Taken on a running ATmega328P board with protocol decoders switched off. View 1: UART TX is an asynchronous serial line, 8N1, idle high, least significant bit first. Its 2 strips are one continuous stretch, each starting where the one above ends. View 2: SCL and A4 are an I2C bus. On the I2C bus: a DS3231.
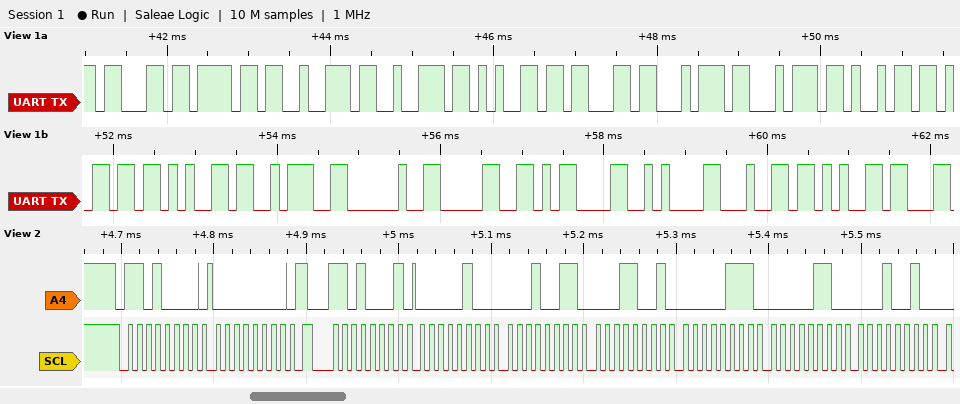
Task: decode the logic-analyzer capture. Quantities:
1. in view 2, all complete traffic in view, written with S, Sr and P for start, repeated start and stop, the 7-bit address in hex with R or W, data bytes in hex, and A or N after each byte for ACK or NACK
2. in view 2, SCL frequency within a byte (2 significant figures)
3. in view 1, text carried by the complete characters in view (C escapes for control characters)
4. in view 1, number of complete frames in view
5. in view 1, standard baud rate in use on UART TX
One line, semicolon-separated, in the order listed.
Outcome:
S 68W A 00 A Sr 68R A 04 A 13 A 19 A 07 A 06 A 12 A; 100 kHz; "correcttime: 0\r\nde"; 18; 9600 baud
